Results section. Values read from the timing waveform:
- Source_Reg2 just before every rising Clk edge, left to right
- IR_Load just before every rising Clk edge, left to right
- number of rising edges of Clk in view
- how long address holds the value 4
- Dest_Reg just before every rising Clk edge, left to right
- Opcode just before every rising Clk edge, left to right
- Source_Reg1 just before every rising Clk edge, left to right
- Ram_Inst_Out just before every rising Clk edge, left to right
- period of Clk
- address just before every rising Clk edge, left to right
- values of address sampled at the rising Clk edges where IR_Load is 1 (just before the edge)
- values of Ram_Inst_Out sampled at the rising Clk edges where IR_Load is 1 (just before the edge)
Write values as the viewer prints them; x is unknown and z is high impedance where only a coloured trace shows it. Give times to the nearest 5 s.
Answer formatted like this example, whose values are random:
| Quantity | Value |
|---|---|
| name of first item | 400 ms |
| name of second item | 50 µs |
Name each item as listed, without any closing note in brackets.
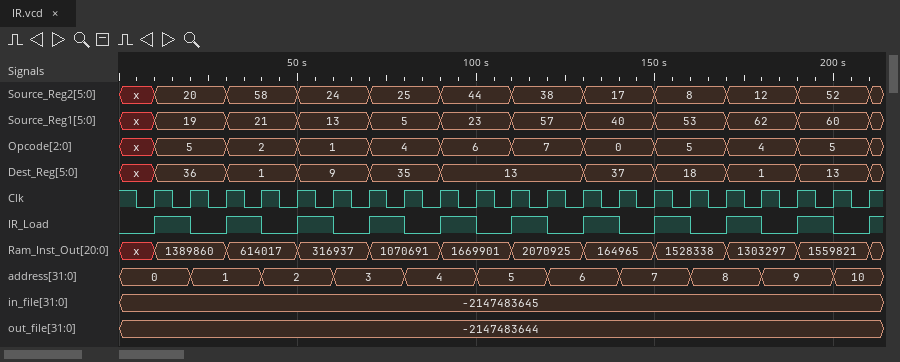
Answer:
| Quantity | Value |
|---|---|
| Source_Reg2 just before every rising Clk edge, left to right | x, 20, 20, 58, 58, 24, 24, 25, 25, 44, 44, 38, 38, 17, 17, 8, 8, 12, 12, 52, 52 |
| IR_Load just before every rising Clk edge, left to right | 0 1 0 1 0 1 0 1 0 1 0 1 0 1 0 1 0 1 0 1 0 |
| number of rising edges of Clk in view | 21 |
| how long address holds the value 4 | 20 s |
| Dest_Reg just before every rising Clk edge, left to right | x, 36, 36, 1, 1, 9, 9, 35, 35, 13, 13, 13, 13, 37, 37, 18, 18, 1, 1, 13, 13 |
| Opcode just before every rising Clk edge, left to right | x, 5, 5, 2, 2, 1, 1, 4, 4, 6, 6, 7, 7, 0, 0, 5, 5, 4, 4, 5, 5 |
| Source_Reg1 just before every rising Clk edge, left to right | x, 19, 19, 21, 21, 13, 13, 5, 5, 23, 23, 57, 57, 40, 40, 53, 53, 62, 62, 60, 60 |
| Ram_Inst_Out just before every rising Clk edge, left to right | x, 1389860, 1389860, 614017, 614017, 316937, 316937, 1070691, 1070691, 1669901, 1669901, 2070925, 2070925, 164965, 164965, 1528338, 1528338, 1303297, 1303297, 1559821, 1559821 |
| period of Clk | 10 s |
| address just before every rising Clk edge, left to right | 0, 0, 1, 1, 2, 2, 3, 3, 4, 4, 5, 5, 6, 6, 7, 7, 8, 8, 9, 9, 10 |
| values of address sampled at the rising Clk edges where IR_Load is 1 | 0, 1, 2, 3, 4, 5, 6, 7, 8, 9 |
| values of Ram_Inst_Out sampled at the rising Clk edges where IR_Load is 1 | 1389860, 614017, 316937, 1070691, 1669901, 2070925, 164965, 1528338, 1303297, 1559821 |
